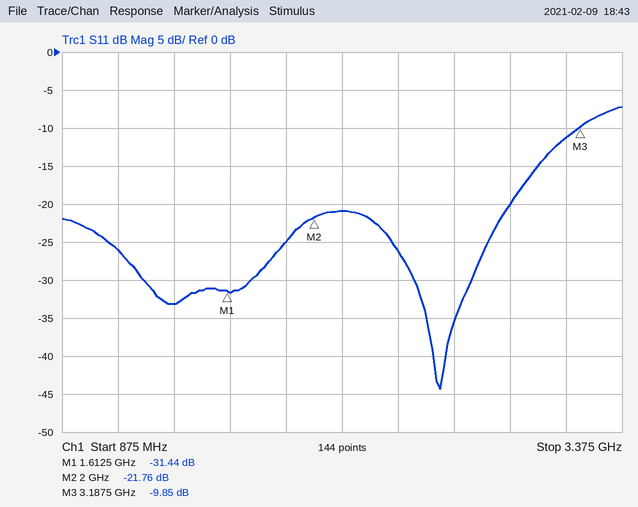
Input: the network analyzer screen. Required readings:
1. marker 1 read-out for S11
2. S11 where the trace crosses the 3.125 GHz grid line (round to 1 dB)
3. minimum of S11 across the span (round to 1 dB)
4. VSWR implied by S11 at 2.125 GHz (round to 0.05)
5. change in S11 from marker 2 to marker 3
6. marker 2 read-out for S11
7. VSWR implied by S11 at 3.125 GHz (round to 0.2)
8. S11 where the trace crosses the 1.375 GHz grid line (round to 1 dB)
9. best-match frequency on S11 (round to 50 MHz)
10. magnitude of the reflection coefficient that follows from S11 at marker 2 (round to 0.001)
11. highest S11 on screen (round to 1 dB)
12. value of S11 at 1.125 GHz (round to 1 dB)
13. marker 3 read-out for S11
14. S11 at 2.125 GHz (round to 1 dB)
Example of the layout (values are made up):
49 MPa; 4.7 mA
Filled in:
-31.44 dB; -11 dB; -44 dB; 1.20; 11.91 dB; -21.76 dB; 1.8; -33 dB; 2.55 GHz; 0.082; -7 dB; -26 dB; -9.85 dB; -21 dB
